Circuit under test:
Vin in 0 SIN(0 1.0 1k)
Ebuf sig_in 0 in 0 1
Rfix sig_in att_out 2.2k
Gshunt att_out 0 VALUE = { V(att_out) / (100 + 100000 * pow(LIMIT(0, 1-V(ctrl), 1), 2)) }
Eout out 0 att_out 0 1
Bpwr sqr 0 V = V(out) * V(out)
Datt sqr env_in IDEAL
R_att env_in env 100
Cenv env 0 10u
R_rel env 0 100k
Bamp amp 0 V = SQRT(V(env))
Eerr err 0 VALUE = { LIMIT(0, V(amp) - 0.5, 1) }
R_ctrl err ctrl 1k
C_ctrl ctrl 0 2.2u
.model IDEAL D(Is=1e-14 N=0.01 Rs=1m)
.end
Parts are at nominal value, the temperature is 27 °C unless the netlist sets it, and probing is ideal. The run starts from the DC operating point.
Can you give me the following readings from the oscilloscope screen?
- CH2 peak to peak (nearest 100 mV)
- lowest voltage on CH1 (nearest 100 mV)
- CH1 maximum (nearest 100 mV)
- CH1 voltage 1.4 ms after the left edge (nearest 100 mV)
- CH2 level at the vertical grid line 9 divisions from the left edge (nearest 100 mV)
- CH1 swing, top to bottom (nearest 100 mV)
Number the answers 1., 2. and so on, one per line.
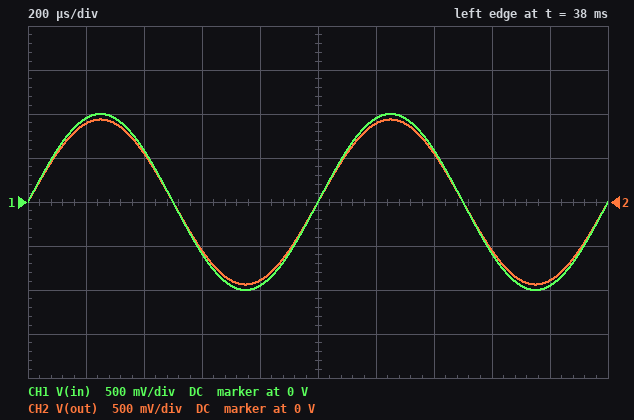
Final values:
1. 1.9 V
2. -1.0 V
3. 1.0 V
4. 600 mV
5. -900 mV
6. 2.0 V
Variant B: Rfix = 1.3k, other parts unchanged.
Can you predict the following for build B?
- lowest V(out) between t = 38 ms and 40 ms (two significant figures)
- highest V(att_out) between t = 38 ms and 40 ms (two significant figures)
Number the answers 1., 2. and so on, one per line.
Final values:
1. -960 mV
2. 960 mV
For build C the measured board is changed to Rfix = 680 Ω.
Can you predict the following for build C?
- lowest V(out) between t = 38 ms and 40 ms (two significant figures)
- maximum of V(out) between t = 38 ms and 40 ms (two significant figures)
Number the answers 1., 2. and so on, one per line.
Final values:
1. -980 mV
2. 980 mV
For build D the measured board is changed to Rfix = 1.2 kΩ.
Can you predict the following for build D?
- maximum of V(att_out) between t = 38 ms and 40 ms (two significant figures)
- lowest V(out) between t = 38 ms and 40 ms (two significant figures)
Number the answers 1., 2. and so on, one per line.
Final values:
1. 960 mV
2. -960 mV
